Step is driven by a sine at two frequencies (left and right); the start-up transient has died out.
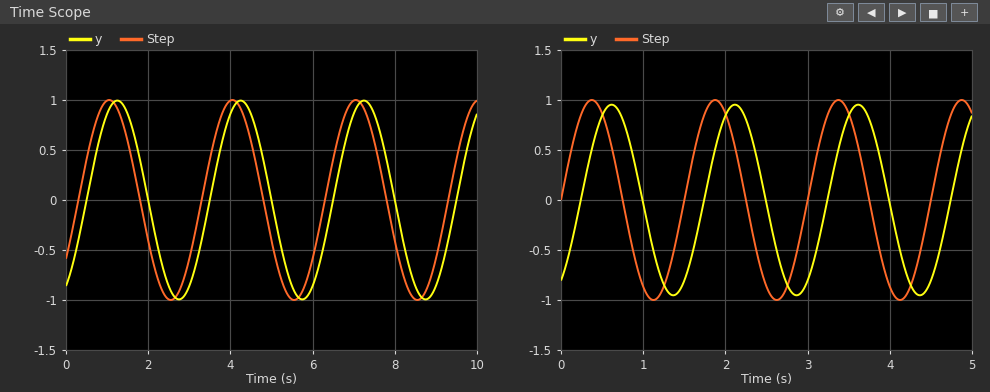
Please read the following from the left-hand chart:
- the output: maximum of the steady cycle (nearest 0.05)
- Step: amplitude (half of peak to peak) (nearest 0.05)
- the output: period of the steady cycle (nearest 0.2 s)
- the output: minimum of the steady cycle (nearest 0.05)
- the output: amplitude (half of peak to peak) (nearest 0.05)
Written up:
1.00
1.00
3.0 s
-1.00
1.00
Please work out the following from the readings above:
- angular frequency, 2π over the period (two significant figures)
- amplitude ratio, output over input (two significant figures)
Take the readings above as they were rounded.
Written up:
2.1 rad/s
1.0
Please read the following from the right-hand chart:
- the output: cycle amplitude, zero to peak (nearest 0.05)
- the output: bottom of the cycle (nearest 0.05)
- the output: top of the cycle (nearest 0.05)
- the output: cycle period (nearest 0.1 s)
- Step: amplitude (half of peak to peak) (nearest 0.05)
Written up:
0.95
-0.95
0.95
1.5 s
1.00
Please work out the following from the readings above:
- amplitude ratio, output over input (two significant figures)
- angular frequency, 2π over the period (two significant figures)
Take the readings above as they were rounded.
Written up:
0.95
4.2 rad/s
